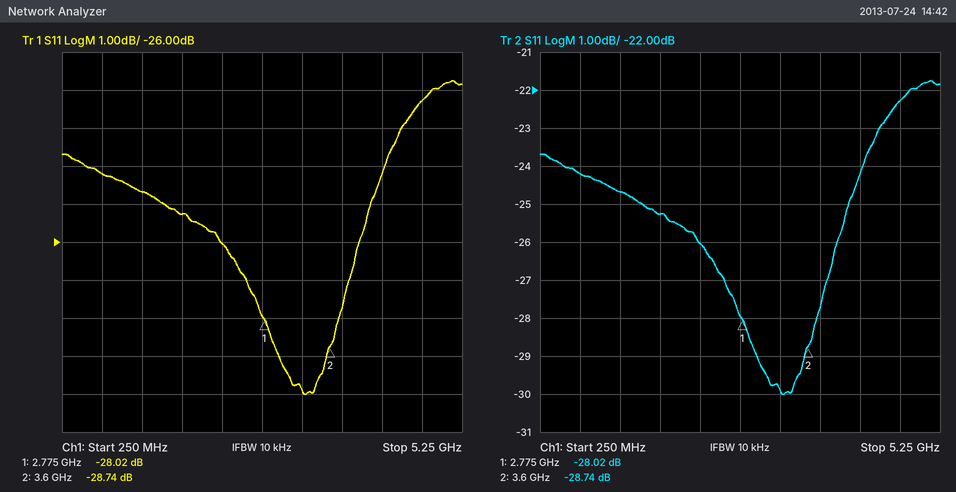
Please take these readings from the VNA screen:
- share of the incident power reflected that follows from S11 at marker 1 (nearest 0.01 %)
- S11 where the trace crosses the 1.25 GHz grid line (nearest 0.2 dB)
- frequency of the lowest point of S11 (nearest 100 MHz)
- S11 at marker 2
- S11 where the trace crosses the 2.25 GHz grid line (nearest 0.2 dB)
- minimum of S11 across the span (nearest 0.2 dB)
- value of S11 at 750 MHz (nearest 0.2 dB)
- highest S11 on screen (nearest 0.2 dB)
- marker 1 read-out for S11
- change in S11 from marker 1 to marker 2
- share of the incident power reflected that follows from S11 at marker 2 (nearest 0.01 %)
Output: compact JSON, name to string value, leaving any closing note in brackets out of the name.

{"share of the incident power reflected that follows from S11 at marker 1": "0.16 %", "S11 where the trace crosses the 1.25 GHz grid line": "-24.6 dB", "frequency of the lowest point of S11": "3.3 GHz", "S11 at marker 2": "-28.74 dB", "S11 where the trace crosses the 2.25 GHz grid line": "-26.0 dB", "minimum of S11 across the span": "-30.0 dB", "value of S11 at 750 MHz": "-24.2 dB", "highest S11 on screen": "-21.8 dB", "marker 1 read-out for S11": "-28.02 dB", "change in S11 from marker 1 to marker 2": "-0.72 dB", "share of the incident power reflected that follows from S11 at marker 2": "0.13 %"}
